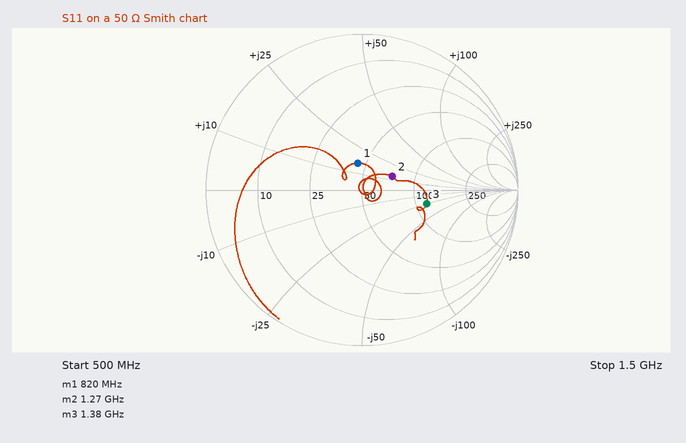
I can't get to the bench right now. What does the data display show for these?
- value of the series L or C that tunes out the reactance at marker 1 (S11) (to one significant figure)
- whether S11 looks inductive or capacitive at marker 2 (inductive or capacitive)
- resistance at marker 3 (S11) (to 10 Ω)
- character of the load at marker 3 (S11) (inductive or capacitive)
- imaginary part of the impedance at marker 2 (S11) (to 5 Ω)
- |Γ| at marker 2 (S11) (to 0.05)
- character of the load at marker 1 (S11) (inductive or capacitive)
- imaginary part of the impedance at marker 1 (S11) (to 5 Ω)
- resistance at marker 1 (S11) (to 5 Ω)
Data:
10 pF
inductive
120 Ω
capacitive
+15 Ω
0.20
inductive
+15 Ω
45 Ω
